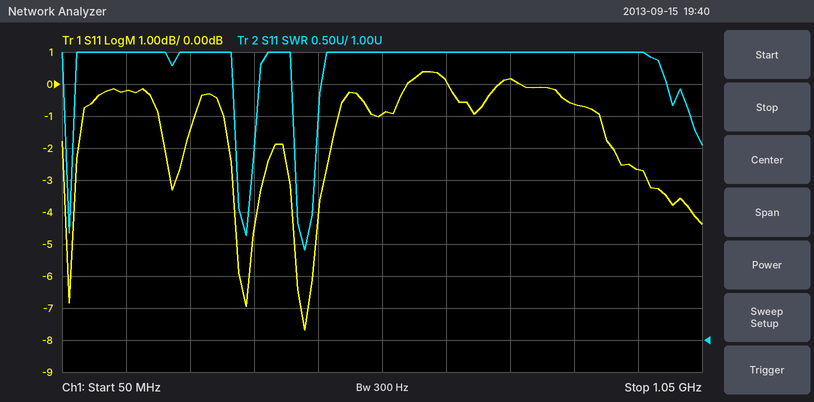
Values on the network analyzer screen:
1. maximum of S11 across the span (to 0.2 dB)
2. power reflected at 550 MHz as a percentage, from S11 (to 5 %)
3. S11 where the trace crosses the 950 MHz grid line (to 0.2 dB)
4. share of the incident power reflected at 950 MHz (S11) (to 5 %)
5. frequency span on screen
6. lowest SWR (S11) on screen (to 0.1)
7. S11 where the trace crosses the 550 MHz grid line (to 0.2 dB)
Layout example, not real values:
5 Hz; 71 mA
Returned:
0.4 dB; 80 %; -2.6 dB; 55 %; 1 GHz; 2.4; -1.0 dB
